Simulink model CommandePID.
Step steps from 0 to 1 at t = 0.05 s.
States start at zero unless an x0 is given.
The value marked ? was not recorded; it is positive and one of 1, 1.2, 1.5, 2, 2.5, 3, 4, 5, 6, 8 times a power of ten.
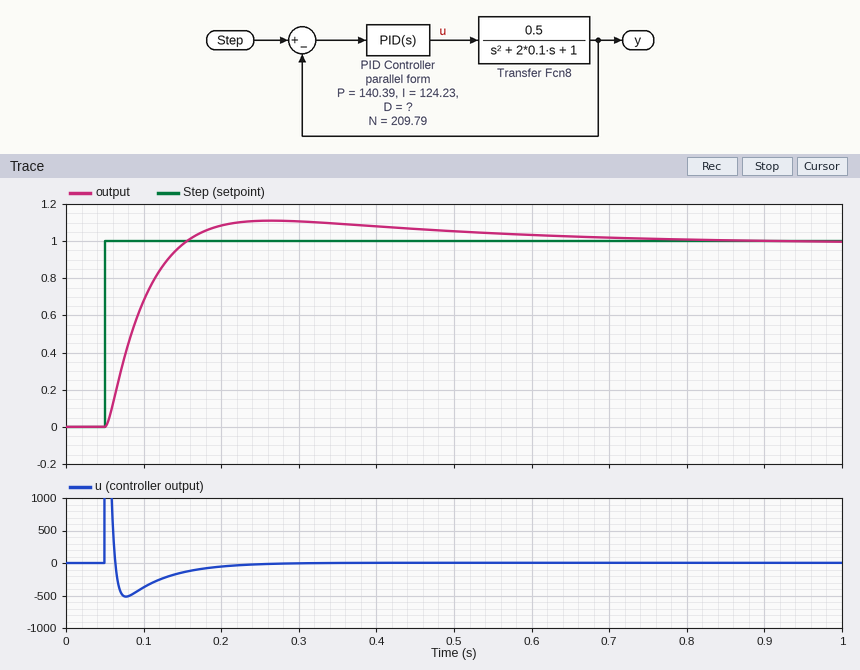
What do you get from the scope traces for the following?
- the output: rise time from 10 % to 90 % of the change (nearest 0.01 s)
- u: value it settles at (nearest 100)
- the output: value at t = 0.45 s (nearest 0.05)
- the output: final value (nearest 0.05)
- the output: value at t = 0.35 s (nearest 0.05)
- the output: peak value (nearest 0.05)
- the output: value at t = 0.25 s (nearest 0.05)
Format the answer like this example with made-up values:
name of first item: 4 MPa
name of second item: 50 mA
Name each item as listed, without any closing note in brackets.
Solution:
the output: rise time from 10 % to 90 % of the change: 0.07 s
u: value it settles at: 0
the output: value at t = 0.45 s: 1.05
the output: final value: 1.00
the output: value at t = 0.35 s: 1.10
the output: peak value: 1.10
the output: value at t = 0.25 s: 1.10
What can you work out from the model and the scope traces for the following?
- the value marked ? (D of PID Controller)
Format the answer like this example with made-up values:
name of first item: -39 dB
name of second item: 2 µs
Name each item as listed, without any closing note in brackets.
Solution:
the value marked ?: 40
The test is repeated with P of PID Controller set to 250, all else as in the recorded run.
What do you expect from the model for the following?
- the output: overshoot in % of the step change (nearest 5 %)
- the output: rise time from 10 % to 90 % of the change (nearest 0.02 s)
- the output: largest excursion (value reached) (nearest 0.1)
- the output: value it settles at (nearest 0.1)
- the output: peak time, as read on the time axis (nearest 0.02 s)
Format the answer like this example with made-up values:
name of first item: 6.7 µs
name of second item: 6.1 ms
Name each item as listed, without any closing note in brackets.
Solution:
the output: overshoot in % of the step change: 15 %
the output: rise time from 10 % to 90 % of the change: 0.06 s
the output: largest excursion (value reached): 1.2
the output: value it settles at: 1.0
the output: peak time, as read on the time axis: 0.22 s
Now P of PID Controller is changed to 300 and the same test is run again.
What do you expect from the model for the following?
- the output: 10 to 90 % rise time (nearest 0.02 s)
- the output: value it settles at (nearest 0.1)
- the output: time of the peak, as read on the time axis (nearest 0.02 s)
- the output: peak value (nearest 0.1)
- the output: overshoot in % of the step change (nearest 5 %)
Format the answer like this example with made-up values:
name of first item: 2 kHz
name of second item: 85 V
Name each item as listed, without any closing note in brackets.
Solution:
the output: 10 to 90 % rise time: 0.06 s
the output: value it settles at: 1.0
the output: time of the peak, as read on the time axis: 0.22 s
the output: peak value: 1.2
the output: overshoot in % of the step change: 20 %
